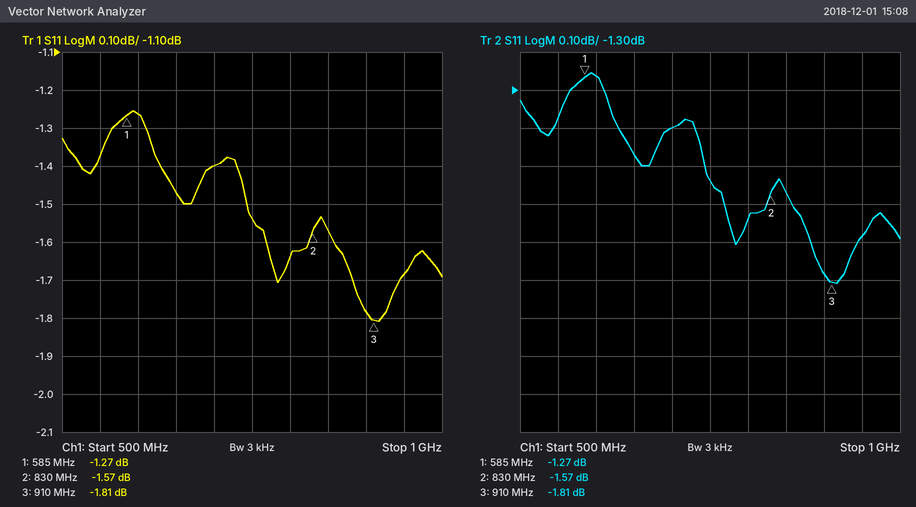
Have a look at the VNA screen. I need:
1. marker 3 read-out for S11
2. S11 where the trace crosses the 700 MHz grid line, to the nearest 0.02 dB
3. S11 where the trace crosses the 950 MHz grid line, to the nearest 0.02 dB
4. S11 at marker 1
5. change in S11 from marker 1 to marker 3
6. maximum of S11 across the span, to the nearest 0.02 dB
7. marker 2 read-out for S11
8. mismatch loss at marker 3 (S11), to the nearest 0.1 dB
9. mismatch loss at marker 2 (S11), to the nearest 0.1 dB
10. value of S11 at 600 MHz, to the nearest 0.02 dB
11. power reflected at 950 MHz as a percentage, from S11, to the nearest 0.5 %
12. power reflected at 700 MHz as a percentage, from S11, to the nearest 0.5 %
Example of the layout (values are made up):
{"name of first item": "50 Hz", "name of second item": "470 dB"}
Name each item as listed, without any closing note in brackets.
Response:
{"marker 3 read-out for S11": "-1.81 dB", "S11 where the trace crosses the 700 MHz grid line, to the nearest 0.02 dB": "-1.40 dB", "S11 where the trace crosses the 950 MHz grid line, to the nearest 0.02 dB": "-1.68 dB", "S11 at marker 1": "-1.27 dB", "change in S11 from marker 1 to marker 3": "-0.54 dB", "maximum of S11 across the span, to the nearest 0.02 dB": "-1.26 dB", "marker 2 read-out for S11": "-1.57 dB", "mismatch loss at marker 3 (S11), to the nearest 0.1 dB": "4.7 dB", "mismatch loss at marker 2 (S11), to the nearest 0.1 dB": "5.2 dB", "value of S11 at 600 MHz, to the nearest 0.02 dB": "-1.26 dB", "power reflected at 950 MHz as a percentage, from S11, to the nearest 0.5 %": "68.0 %", "power reflected at 700 MHz as a percentage, from S11, to the nearest 0.5 %": "72.5 %"}
